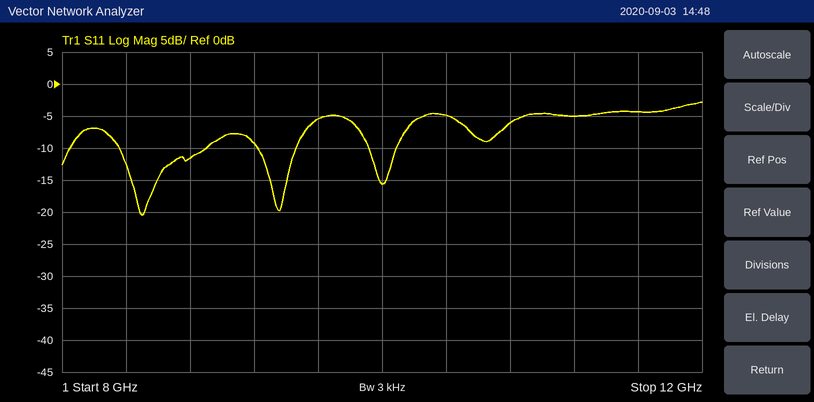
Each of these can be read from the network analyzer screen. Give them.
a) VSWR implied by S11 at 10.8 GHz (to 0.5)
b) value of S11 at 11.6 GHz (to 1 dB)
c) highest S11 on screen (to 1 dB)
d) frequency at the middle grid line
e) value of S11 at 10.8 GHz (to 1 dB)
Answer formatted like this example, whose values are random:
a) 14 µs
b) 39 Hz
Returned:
a) 3.0
b) -4 dB
c) -3 dB
d) 10 GHz
e) -6 dB
